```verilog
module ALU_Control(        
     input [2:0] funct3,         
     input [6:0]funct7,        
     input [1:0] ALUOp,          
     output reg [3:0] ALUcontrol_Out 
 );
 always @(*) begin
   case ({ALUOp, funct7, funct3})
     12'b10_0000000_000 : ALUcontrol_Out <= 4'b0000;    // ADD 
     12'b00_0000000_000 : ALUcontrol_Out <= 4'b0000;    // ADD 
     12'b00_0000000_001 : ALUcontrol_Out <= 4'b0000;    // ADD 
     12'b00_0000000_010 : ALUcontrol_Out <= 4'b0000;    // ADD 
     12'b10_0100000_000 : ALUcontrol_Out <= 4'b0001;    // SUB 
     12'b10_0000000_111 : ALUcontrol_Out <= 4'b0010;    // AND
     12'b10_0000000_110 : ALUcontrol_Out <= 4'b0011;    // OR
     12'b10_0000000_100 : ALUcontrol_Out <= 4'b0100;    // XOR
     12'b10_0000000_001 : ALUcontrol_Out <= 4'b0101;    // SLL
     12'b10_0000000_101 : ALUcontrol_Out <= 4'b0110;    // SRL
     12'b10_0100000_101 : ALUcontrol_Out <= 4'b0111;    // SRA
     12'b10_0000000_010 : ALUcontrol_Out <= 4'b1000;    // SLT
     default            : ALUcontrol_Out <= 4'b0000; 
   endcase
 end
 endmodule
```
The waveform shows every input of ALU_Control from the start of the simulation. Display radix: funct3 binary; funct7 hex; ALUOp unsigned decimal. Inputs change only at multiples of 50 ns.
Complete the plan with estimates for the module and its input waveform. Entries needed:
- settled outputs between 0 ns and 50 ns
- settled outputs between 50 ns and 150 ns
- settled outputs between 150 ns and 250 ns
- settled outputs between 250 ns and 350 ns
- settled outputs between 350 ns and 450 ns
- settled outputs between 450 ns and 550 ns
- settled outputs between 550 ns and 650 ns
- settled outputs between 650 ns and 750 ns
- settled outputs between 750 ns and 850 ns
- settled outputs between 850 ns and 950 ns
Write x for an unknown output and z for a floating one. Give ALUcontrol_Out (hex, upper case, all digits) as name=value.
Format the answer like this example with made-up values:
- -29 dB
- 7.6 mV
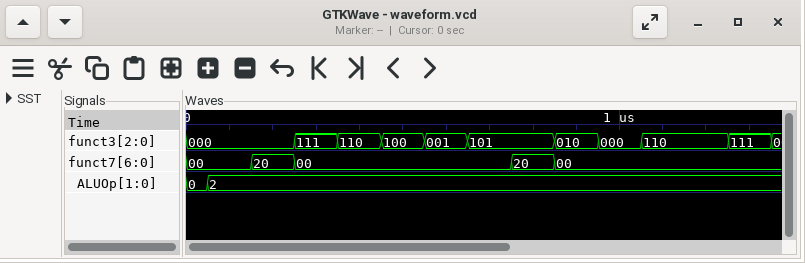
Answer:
- ALUcontrol_Out=0
- ALUcontrol_Out=0
- ALUcontrol_Out=1
- ALUcontrol_Out=2
- ALUcontrol_Out=3
- ALUcontrol_Out=4
- ALUcontrol_Out=5
- ALUcontrol_Out=6
- ALUcontrol_Out=7
- ALUcontrol_Out=8
